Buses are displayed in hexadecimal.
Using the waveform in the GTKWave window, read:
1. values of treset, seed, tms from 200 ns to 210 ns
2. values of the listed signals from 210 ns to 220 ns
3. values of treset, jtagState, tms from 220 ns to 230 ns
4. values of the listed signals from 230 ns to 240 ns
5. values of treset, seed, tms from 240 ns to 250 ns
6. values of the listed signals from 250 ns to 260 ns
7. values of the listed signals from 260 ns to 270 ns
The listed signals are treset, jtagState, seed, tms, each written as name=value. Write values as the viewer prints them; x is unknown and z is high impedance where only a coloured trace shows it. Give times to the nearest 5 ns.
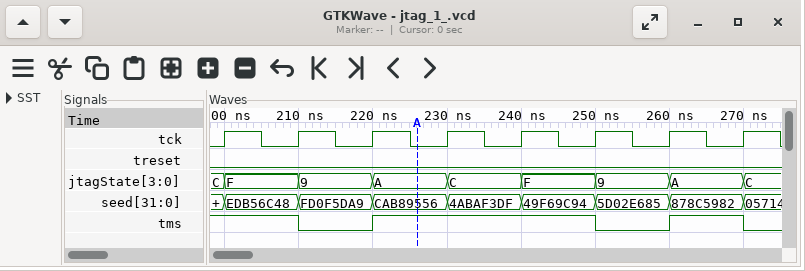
treset=0, seed=EDB56C48, tms=1
treset=0, jtagState=9, seed=FD0F5DA9, tms=0
treset=0, jtagState=A, tms=1
treset=0, jtagState=C, seed=4ABAF3DF, tms=1
treset=0, seed=49F69C94, tms=1
treset=0, jtagState=9, seed=5D02E685, tms=0
treset=0, jtagState=A, seed=878C5982, tms=1
